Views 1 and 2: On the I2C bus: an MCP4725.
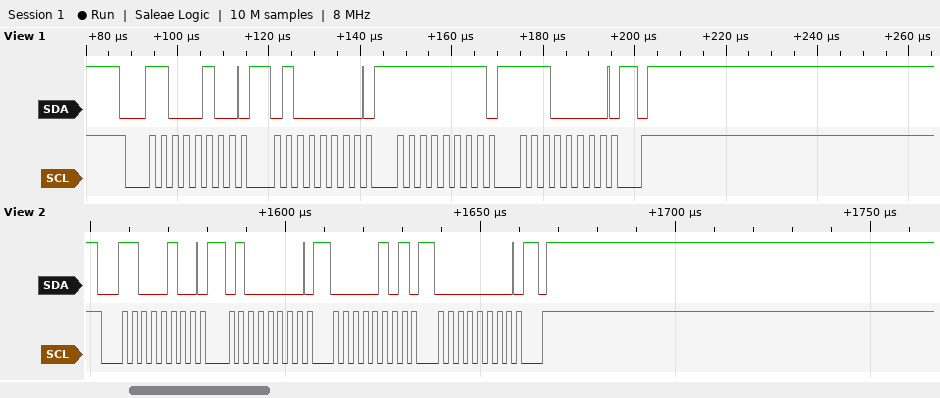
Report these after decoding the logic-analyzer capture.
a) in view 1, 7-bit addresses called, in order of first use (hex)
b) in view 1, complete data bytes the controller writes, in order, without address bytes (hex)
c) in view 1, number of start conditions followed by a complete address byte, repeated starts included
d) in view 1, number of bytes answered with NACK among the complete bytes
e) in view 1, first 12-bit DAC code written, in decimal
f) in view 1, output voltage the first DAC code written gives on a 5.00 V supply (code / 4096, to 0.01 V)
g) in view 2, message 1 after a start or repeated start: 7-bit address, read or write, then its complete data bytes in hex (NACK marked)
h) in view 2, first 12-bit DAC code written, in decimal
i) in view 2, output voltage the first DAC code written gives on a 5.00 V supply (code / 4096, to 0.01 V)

0x62
40 FF E0
1
0
4094
5.00 V
0x62 write: 40 05 00
80
0.10 V
